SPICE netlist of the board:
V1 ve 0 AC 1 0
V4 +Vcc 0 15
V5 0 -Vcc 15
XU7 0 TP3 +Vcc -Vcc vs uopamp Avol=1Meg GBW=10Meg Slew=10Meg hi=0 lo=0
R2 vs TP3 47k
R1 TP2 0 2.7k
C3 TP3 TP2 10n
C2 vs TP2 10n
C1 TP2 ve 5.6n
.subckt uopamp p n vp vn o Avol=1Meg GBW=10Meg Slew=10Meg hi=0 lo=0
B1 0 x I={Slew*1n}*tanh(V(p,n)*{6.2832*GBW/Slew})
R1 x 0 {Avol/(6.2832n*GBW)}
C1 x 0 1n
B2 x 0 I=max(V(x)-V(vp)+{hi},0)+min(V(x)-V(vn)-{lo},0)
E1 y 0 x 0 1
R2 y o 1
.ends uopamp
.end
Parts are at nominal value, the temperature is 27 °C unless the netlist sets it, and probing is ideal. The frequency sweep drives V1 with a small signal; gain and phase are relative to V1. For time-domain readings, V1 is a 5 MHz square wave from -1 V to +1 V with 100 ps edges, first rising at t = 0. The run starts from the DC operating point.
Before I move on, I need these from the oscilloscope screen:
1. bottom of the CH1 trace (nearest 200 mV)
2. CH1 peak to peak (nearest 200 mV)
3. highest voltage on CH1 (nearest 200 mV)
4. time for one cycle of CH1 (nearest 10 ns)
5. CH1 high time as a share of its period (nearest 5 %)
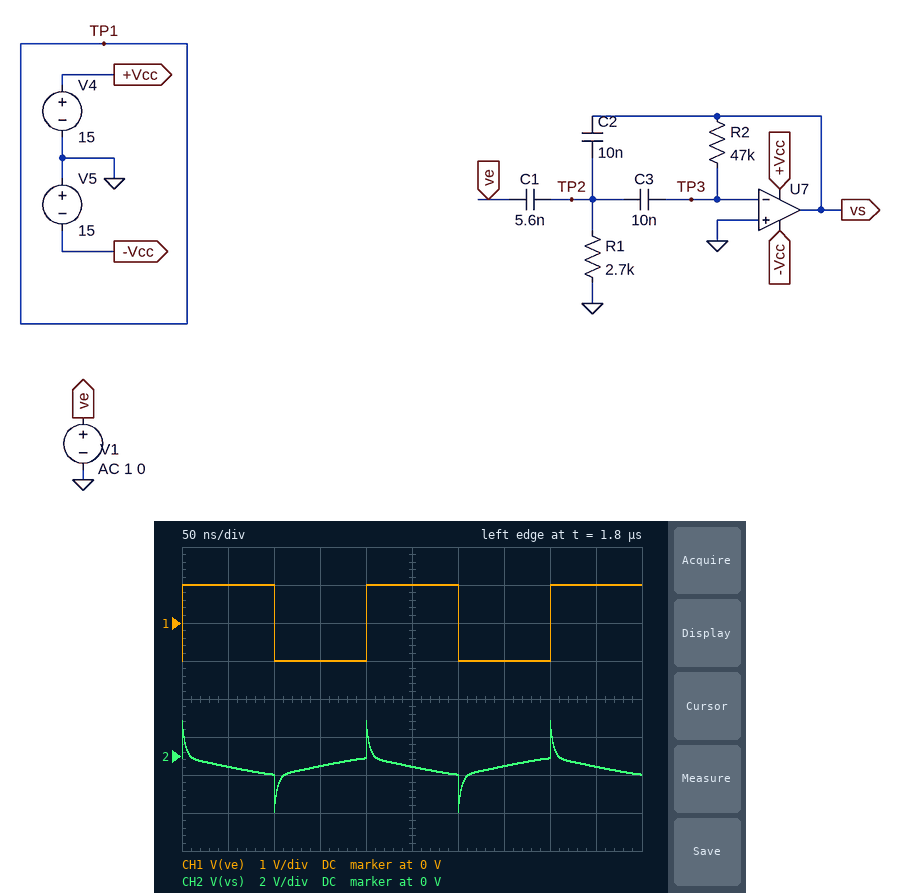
-1.0 V
2.0 V
1.0 V
200 ns
50 %
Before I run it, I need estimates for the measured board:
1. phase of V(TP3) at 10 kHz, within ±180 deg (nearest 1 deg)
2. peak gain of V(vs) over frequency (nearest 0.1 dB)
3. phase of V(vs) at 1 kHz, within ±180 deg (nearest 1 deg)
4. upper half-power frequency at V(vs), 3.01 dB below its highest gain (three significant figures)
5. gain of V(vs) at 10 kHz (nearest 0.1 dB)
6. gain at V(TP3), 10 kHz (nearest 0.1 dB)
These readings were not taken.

95 deg
-0.4 dB
-41 deg
2.96 kHz
-4.9 dB
-64.9 dB
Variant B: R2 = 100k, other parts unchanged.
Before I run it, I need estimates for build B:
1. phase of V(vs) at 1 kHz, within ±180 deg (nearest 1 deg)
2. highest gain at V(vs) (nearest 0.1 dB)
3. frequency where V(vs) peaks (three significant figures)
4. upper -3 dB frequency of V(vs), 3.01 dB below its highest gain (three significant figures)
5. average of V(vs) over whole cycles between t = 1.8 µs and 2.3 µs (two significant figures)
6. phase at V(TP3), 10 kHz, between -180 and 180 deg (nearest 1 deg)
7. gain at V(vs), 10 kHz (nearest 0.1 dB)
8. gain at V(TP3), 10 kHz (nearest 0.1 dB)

-99 deg
2.7 dB
1.01 kHz
1.37 kHz
-560 mV
92 deg
-5.0 dB
-65.0 dB
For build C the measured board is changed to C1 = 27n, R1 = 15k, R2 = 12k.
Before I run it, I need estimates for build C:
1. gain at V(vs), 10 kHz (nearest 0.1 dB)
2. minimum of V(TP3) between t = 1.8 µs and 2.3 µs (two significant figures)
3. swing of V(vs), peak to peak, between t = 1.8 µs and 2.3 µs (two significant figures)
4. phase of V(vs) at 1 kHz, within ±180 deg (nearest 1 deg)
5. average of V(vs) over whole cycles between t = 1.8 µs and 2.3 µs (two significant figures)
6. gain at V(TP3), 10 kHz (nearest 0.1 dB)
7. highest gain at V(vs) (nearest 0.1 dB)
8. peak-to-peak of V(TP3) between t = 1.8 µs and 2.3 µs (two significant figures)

7.3 dB
-1.0 V
4.9 V
-86 deg
-1.2 V
-52.7 dB
8.6 dB
2.8 V
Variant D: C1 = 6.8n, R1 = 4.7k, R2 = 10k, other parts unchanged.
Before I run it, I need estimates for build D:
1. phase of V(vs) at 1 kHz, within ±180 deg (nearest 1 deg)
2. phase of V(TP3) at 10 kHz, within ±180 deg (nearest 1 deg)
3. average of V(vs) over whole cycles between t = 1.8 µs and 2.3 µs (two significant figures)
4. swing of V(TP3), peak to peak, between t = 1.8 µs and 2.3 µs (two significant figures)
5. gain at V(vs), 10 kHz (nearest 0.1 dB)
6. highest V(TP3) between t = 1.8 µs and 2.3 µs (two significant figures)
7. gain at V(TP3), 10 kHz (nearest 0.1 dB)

-44 deg
114 deg
-650 mV
3.7 V
-3.7 dB
1.8 V
-63.7 dB
